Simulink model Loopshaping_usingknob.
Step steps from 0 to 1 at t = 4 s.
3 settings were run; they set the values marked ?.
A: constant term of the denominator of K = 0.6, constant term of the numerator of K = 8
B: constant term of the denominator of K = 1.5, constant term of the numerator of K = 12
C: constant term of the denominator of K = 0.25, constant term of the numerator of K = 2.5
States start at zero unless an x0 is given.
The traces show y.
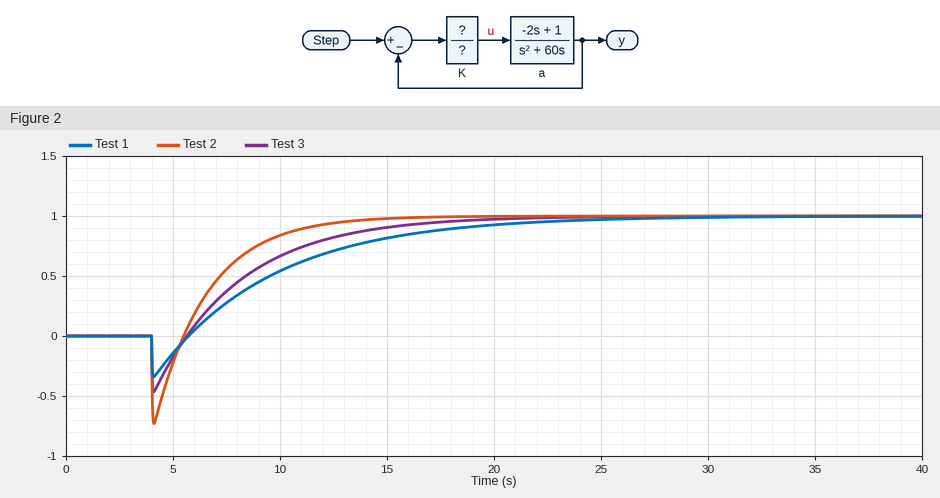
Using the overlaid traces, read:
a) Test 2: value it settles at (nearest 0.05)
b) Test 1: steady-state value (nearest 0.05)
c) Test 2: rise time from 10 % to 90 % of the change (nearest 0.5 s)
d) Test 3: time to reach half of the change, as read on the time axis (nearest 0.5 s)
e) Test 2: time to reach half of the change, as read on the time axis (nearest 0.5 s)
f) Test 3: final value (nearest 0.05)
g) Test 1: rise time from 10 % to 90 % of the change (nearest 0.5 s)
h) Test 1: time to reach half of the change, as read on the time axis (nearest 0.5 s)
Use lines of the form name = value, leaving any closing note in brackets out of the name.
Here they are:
Test 2: value it settles at = 1.00
Test 1: steady-state value = 1.00
Test 2: rise time from 10 % to 90 % of the change = 5.5 s
Test 3: time to reach half of the change, as read on the time axis = 8.5 s
Test 2: time to reach half of the change, as read on the time axis = 7.0 s
Test 3: final value = 1.00
Test 1: rise time from 10 % to 90 % of the change = 12.0 s
Test 1: time to reach half of the change, as read on the time axis = 9.5 s
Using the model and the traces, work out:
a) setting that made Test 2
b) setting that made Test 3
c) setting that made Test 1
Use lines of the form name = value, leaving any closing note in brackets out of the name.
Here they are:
setting that made Test 2 = A
setting that made Test 3 = C
setting that made Test 1 = B
